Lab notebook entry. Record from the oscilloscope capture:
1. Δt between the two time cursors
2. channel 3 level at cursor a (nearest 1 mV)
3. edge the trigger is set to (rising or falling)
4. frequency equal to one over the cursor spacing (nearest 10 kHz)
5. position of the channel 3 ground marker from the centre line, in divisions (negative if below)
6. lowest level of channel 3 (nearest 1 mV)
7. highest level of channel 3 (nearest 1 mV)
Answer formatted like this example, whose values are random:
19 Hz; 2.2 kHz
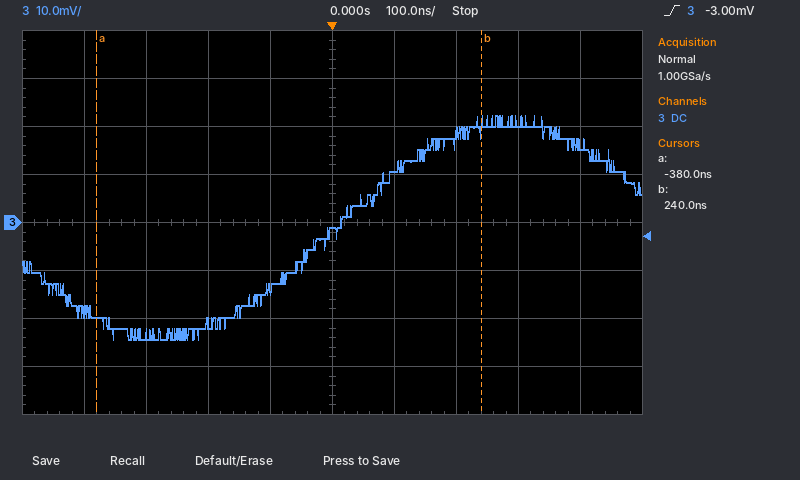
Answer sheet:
620 ns; -20 mV; rising; 1.61 MHz; 0.0 div; -24 mV; 22 mV
